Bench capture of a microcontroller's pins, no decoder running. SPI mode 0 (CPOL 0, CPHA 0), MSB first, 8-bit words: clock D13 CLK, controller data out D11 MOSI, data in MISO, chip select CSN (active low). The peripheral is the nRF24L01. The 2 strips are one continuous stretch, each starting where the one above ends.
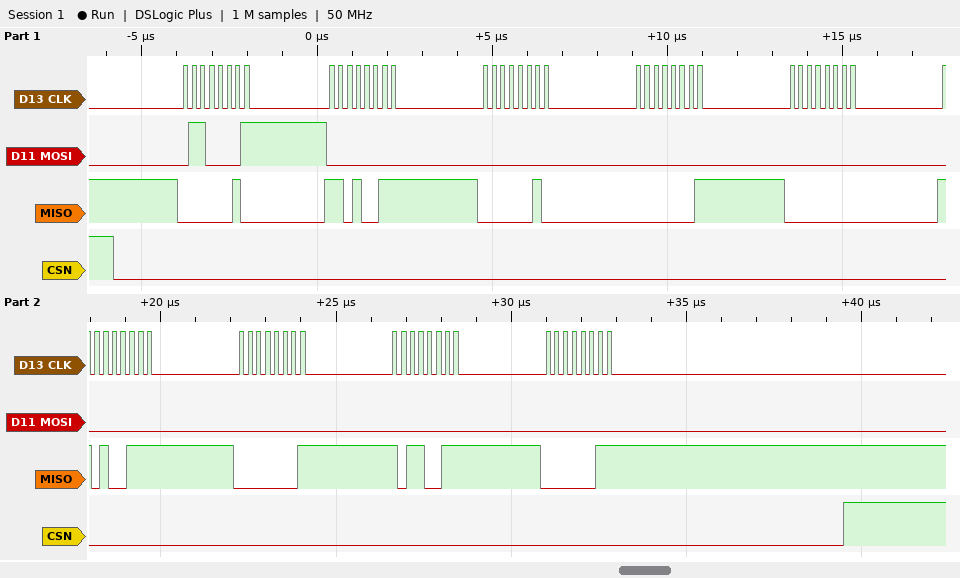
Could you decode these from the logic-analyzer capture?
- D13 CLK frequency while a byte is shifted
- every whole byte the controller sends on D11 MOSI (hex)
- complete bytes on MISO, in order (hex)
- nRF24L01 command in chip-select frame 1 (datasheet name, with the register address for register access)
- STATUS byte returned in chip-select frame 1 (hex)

4 MHz
61 00 00 00 00 00 00 00 00
02 D3 02 01 00 A7 01 B3 03
R_RX_PAYLOAD
0x02
